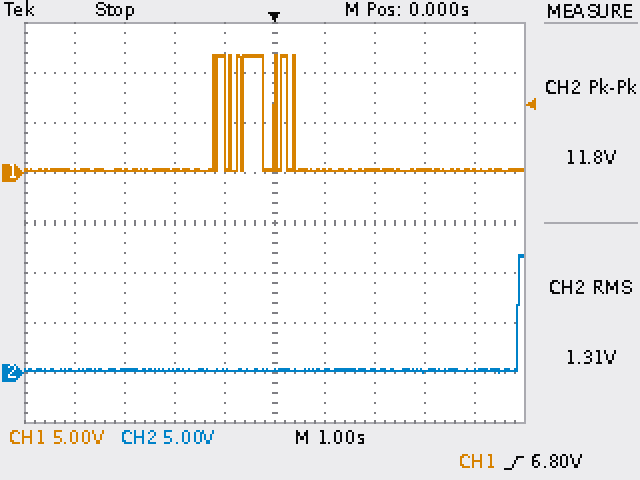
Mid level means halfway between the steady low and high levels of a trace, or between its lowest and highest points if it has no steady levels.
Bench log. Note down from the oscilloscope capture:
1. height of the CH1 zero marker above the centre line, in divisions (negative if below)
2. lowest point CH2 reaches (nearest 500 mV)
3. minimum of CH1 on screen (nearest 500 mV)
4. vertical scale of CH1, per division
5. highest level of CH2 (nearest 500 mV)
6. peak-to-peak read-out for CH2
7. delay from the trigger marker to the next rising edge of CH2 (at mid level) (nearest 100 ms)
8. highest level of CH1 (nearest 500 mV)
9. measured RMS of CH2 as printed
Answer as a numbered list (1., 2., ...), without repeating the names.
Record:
1. +1.0 div
2. 0.0 V
3. 0.0 V
4. 5 V
5. 12.0 V
6. 11.8 V
7. 4.9 s
8. 12.0 V
9. 1.31 V
